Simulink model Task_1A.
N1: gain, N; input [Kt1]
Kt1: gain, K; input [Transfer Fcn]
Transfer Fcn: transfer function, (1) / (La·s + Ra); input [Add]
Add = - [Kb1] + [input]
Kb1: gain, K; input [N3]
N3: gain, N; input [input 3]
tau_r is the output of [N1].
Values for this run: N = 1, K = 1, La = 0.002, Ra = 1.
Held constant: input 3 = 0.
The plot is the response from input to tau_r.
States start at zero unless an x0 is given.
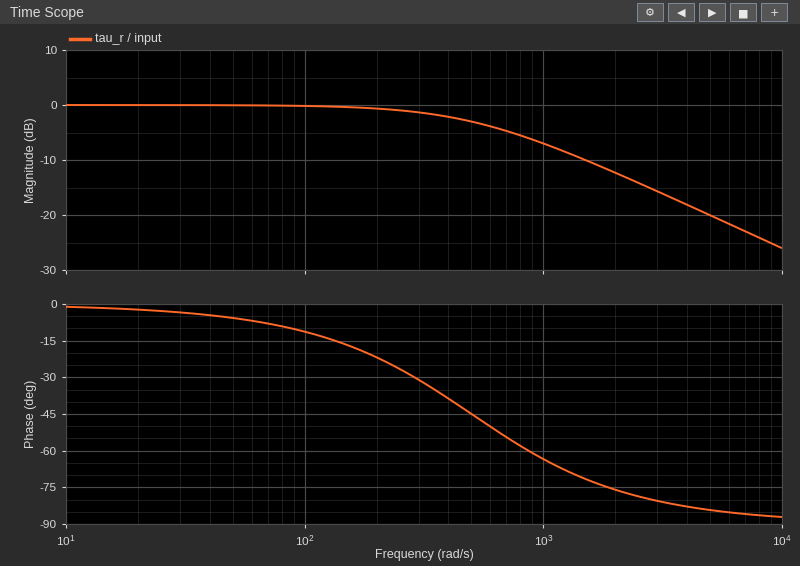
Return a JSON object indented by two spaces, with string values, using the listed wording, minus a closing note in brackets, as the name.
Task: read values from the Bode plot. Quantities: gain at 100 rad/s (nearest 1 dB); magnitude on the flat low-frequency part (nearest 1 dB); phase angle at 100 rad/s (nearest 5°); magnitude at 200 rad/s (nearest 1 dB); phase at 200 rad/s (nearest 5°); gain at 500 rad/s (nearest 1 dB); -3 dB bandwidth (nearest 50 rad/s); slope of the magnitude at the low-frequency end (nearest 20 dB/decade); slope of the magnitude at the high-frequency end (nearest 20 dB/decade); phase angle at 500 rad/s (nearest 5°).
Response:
{
  "gain at 100 rad/s": "0 dB",
  "magnitude on the flat low-frequency part": "0 dB",
  "phase angle at 100 rad/s": "-10°",
  "magnitude at 200 rad/s": "-1 dB",
  "phase at 200 rad/s": "-20°",
  "gain at 500 rad/s": "-3 dB",
  "-3 dB bandwidth": "500 rad/s",
  "slope of the magnitude at the low-frequency end": "0 dB/decade",
  "slope of the magnitude at the high-frequency end": "-20 dB/decade",
  "phase angle at 500 rad/s": "-45°"
}
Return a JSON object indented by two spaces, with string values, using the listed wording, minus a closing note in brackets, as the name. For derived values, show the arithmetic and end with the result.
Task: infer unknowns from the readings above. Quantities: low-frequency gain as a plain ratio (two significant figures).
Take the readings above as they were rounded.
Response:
{
  "low-frequency gain as a plain ratio": "10^(0 / 20) = 1.0"
}
